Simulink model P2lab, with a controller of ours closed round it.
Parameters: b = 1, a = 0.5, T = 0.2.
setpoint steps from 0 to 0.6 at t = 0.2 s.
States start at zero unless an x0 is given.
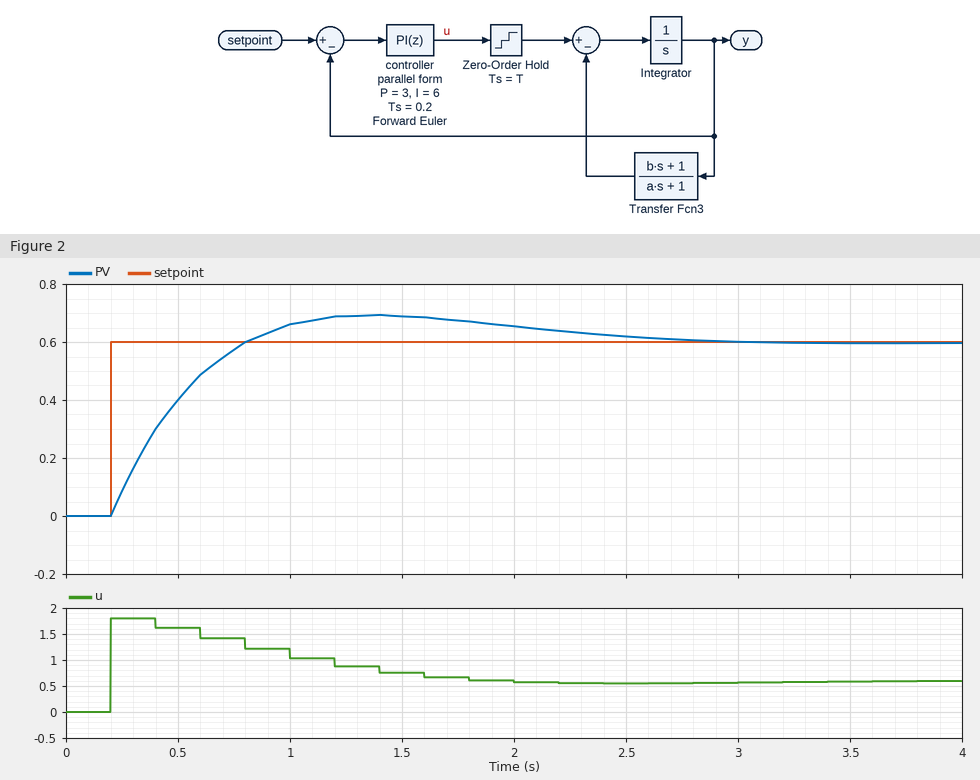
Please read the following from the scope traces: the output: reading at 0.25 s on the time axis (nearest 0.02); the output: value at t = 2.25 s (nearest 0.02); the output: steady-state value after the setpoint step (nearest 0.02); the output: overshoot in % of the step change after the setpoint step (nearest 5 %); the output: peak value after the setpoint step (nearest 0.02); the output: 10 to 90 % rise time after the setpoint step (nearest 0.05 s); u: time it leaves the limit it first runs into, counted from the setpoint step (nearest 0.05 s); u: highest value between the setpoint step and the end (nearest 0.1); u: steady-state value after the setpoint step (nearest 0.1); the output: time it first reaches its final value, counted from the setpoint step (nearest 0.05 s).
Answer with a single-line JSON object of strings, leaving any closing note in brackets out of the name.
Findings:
{"the output: reading at 0.25 s on the time axis": "0.08", "the output: value at t = 2.25 s": "0.64", "the output: steady-state value after the setpoint step": "0.60", "the output: overshoot in % of the step change after the setpoint step": "15 %", "the output: peak value after the setpoint step": "0.70", "the output: 10 to 90 % rise time after the setpoint step": "0.45 s", "u: time it leaves the limit it first runs into, counted from the setpoint step": "0.20 s", "u: highest value between the setpoint step and the end": "1.8", "u: steady-state value after the setpoint step": "0.6", "the output: time it first reaches its final value, counted from the setpoint step": "0.60 s"}
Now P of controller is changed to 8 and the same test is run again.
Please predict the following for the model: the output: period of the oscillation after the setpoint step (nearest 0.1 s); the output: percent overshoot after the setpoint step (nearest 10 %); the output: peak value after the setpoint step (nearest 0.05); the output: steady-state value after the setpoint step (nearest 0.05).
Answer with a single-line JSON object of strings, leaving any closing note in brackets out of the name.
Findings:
{"the output: period of the oscillation after the setpoint step": "0.4 s", "the output: percent overshoot after the setpoint step": "30 %", "the output: peak value after the setpoint step": "0.80", "the output: steady-state value after the setpoint step": "0.60"}
